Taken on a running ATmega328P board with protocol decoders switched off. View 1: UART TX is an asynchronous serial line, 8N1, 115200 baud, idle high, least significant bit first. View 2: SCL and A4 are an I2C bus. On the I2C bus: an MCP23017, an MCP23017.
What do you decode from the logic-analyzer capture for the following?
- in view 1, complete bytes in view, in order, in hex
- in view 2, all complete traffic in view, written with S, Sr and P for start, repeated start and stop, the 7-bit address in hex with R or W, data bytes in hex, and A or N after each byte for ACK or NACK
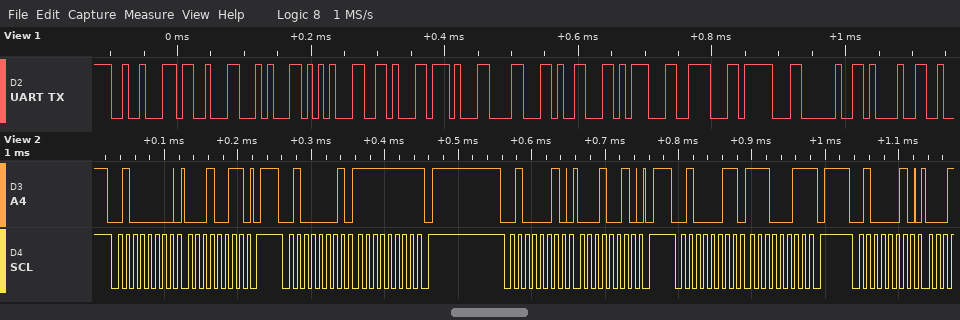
12 13 14 15 16 17 18 19 1D 1E 1F 20 21
S 20W A 13 A P S 20R A FF N P S 21W A 12 A P S 21R A E3 N P S 21W A
